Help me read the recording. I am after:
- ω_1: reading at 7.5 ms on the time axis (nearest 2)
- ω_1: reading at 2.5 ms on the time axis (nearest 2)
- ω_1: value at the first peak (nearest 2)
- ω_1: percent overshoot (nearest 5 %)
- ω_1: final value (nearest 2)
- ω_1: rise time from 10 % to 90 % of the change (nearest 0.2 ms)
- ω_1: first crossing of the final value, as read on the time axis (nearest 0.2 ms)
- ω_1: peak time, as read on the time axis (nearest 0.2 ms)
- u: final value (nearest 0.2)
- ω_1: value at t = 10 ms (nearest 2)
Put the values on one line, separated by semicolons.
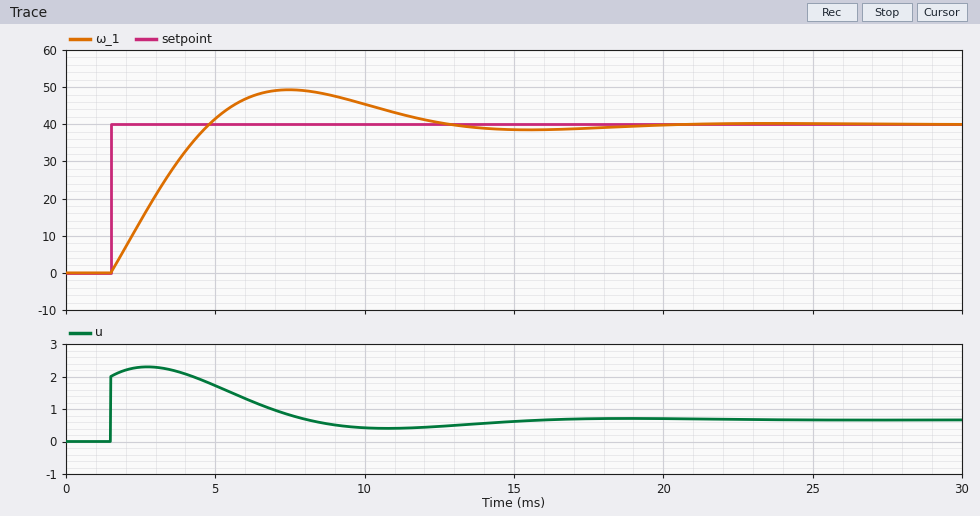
50; 14; 50; 25 %; 40; 2.6 ms; 4.8 ms; 7.4 ms; 0.6; 46
